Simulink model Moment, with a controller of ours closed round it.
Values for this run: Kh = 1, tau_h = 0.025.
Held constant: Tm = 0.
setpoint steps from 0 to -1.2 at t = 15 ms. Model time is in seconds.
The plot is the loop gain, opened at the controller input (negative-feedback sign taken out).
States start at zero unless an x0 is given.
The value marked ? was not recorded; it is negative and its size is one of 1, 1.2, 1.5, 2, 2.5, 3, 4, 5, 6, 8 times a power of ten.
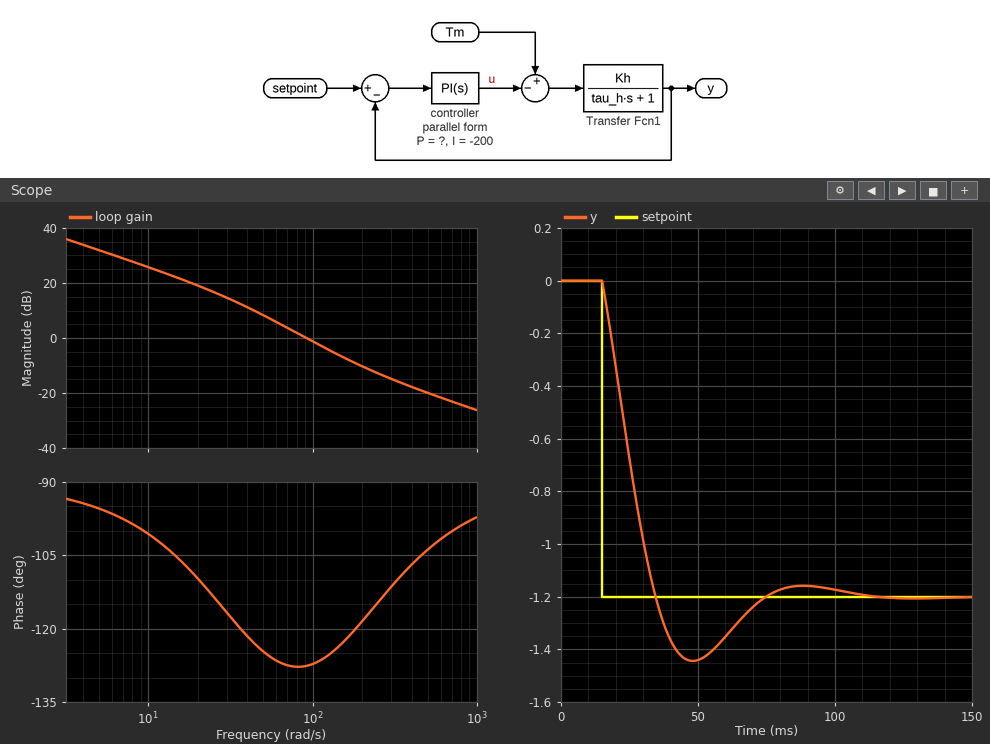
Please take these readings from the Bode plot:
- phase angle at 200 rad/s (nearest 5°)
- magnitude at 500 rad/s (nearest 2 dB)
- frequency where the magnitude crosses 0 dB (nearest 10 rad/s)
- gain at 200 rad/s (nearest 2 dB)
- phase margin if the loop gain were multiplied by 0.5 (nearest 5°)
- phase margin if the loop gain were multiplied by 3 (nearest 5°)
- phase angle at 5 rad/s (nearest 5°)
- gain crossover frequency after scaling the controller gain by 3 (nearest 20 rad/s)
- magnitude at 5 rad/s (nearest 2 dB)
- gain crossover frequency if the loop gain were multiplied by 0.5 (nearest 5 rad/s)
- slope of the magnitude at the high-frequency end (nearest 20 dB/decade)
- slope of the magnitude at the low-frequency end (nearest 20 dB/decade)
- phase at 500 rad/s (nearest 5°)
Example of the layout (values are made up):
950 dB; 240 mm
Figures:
-120°; -20 dB; 90 rad/s; -10 dB; 55°; 60°; -95°; 180 rad/s; 32 dB; 60 rad/s; -20 dB/decade; -20 dB/decade; -105°
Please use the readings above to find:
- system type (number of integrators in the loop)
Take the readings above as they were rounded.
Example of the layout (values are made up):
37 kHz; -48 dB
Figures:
1
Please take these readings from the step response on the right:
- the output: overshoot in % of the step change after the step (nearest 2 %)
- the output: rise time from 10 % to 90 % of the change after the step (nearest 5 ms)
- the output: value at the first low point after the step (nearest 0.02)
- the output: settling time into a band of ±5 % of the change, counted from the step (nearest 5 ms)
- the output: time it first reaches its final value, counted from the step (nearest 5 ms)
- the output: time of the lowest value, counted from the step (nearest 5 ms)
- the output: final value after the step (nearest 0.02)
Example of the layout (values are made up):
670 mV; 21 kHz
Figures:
20 %; 15 ms; -1.44; 55 ms; 20 ms; 35 ms; -1.20
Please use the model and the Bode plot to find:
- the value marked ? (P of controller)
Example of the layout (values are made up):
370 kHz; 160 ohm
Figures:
-1.2
